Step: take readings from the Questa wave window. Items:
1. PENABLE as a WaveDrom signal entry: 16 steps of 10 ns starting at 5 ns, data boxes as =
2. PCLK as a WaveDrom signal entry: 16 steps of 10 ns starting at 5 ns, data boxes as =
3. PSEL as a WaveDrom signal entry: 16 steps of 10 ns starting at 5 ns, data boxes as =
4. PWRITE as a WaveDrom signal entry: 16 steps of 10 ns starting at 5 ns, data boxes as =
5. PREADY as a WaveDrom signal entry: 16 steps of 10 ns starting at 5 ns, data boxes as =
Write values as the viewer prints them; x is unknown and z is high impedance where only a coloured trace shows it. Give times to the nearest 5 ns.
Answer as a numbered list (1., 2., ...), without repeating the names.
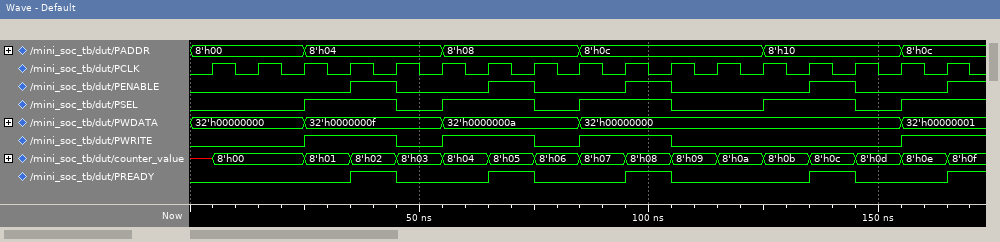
1. {name: 'PENABLE', wave: '0..10.10.10..10.'}
2. {name: 'PCLK', wave: 'p...............'}
3. {name: 'PSEL', wave: '0.1.01.01.0.1.01'}
4. {name: 'PWRITE', wave: '0.1.01.01.0....1'}
5. {name: 'PREADY', wave: '0..10.10.10..10.'}
